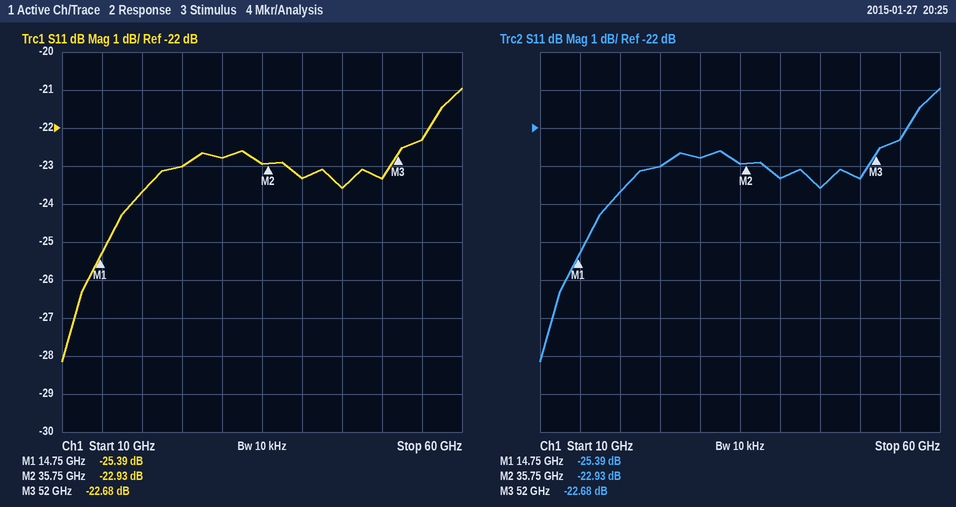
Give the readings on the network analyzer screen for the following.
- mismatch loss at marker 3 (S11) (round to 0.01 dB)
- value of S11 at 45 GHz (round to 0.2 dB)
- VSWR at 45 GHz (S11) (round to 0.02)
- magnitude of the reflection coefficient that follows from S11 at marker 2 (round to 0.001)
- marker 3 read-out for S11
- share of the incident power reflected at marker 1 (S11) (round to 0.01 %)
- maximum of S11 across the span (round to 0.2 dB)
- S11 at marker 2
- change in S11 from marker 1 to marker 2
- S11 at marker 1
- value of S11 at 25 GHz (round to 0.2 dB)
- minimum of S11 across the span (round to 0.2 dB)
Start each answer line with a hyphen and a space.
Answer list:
- 0.02 dB
- -23.6 dB
- 1.14
- 0.071
- -22.68 dB
- 0.29 %
- -21.0 dB
- -22.93 dB
- 2.46 dB
- -25.39 dB
- -23.0 dB
- -28.2 dB
